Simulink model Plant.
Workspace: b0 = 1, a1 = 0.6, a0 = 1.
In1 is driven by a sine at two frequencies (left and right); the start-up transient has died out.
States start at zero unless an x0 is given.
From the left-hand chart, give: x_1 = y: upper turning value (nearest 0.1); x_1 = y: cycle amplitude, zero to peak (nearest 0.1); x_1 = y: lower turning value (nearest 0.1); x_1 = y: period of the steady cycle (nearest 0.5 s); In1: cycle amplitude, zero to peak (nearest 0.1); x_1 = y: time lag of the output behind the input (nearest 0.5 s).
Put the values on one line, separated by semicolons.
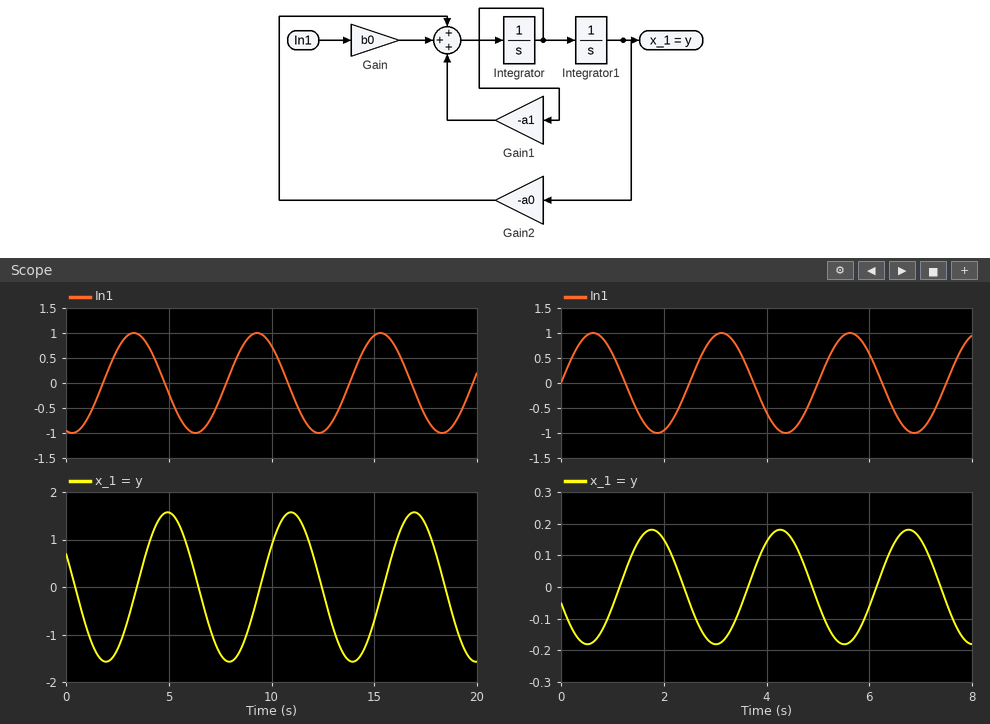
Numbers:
1.6; 1.6; -1.6; 6.0 s; 1.0; 1.5 s
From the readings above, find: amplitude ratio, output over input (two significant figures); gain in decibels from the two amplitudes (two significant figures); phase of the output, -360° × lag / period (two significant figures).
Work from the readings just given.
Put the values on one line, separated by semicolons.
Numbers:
1.6; 4.1 dB; -90°
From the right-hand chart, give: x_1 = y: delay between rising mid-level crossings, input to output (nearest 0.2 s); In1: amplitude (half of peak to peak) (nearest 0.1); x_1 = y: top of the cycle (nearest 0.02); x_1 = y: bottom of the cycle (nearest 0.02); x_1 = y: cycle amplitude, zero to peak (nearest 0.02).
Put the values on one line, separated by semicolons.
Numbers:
1.2 s; 1.0; 0.18; -0.18; 0.18
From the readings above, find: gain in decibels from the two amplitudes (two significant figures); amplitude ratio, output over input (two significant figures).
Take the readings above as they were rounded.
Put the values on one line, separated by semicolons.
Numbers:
-15 dB; 0.18
